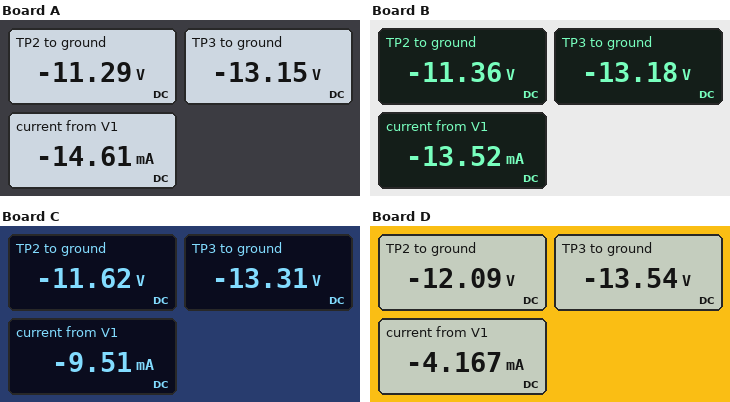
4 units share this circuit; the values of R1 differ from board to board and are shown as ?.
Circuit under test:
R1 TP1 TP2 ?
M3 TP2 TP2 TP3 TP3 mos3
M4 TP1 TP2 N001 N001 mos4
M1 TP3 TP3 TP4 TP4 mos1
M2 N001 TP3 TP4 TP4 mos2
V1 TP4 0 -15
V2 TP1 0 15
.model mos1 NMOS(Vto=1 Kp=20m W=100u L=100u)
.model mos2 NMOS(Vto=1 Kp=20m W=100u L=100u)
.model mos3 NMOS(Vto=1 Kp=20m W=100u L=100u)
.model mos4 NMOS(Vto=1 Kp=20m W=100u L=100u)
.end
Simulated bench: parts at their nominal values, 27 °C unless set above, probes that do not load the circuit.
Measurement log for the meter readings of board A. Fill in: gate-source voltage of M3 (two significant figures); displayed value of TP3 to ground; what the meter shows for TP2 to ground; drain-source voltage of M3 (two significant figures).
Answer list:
1.9 V
-13.15 V
-11.29 V
1.9 V
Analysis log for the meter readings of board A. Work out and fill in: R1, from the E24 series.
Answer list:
3.6 kΩ
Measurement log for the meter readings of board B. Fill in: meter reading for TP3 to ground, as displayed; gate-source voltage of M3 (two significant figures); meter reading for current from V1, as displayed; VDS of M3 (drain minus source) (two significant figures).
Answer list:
-13.18 V
1.8 V
-13.52 mA
1.8 V
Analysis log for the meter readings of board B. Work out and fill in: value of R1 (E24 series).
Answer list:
3.9 kΩ
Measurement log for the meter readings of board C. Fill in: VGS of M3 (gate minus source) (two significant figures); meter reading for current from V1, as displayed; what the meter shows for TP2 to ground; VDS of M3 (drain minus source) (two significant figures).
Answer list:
1.7 V
-9.51 mA
-11.62 V
1.7 V
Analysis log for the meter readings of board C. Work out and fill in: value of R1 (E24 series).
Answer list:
5.6 kΩ
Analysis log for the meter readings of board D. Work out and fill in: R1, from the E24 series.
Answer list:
13 kΩ
